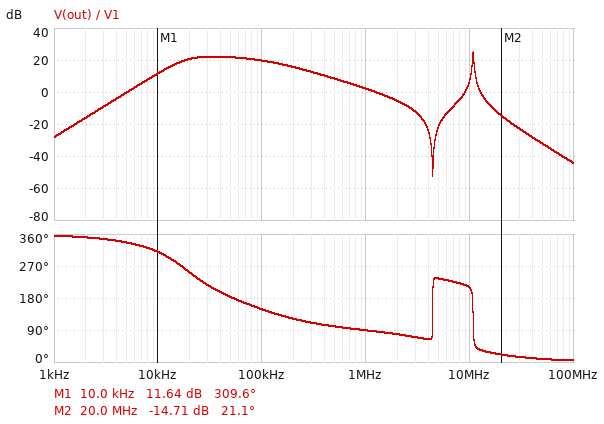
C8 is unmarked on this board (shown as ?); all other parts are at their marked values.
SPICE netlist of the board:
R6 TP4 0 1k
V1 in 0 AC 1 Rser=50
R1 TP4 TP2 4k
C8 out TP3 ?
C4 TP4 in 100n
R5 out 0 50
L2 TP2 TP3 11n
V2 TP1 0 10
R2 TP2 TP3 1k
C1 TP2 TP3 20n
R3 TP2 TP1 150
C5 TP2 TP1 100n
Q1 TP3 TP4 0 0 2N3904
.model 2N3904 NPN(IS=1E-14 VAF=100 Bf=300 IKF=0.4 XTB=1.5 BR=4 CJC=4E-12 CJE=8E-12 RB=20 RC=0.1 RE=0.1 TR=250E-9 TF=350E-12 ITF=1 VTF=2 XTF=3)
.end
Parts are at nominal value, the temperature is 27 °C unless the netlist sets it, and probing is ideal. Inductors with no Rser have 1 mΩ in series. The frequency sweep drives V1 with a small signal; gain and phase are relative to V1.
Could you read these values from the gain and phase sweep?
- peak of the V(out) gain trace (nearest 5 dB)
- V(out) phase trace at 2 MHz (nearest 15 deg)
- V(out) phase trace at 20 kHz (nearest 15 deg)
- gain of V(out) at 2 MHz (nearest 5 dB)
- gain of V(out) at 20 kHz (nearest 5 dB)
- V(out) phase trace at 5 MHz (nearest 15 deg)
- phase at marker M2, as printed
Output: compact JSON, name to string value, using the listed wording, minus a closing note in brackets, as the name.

{"peak of the V(out) gain trace": "25 dB", "V(out) phase trace at 2 MHz": "75 deg", "V(out) phase trace at 20 kHz": "255 deg", "gain of V(out) at 2 MHz": "-5 dB", "gain of V(out) at 20 kHz": "20 dB", "V(out) phase trace at 5 MHz": "240 deg", "phase at marker M2, as printed": "21.1 deg"}
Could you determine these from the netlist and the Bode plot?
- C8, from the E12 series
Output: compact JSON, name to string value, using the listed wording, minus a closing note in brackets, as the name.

{"C8, from the E12 series": "56 nF"}
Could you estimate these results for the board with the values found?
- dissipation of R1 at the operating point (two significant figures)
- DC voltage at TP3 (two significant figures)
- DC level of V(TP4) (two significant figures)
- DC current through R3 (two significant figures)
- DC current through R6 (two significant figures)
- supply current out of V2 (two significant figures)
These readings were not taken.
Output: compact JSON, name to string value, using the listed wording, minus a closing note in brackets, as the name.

{"dissipation of R1 at the operating point": "3.1 mW", "DC voltage at TP3": "4.3 V", "DC level of V(TP4)": "760 mV", "DC current through R3": "38 mA", "DC current through R6": "760 µA", "supply current out of V2": "38 mA"}
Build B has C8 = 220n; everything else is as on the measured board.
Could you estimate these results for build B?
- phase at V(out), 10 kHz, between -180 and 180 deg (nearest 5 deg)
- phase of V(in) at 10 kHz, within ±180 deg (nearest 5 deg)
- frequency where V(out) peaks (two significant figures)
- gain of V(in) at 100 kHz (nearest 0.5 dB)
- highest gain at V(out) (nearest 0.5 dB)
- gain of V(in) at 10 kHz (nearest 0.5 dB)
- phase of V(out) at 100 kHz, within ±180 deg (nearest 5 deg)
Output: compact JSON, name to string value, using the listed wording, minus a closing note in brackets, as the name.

{"phase at V(out), 10 kHz, between -180 and 180 deg": "-85 deg", "phase of V(in) at 10 kHz, within ±180 deg": "-15 deg", "frequency where V(out) peaks": "27 kHz", "gain of V(in) at 100 kHz": "-3.0 dB", "highest gain at V(out)": "25.5 dB", "gain of V(in) at 10 kHz": "-1.5 dB", "phase of V(out) at 100 kHz, within ±180 deg": "130 deg"}
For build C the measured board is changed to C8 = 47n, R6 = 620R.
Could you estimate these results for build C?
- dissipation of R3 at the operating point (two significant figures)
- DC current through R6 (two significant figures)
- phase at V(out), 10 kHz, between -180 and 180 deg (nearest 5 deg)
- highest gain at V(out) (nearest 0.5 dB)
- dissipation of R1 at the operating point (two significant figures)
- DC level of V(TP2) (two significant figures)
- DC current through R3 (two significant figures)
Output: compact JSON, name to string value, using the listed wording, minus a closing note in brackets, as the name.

{"dissipation of R3 at the operating point": "110 mW", "DC current through R6": "1.2 mA", "phase at V(out), 10 kHz, between -180 and 180 deg": "-55 deg", "highest gain at V(out)": "24.5 dB", "dissipation of R1 at the operating point": "6.6 mW", "DC level of V(TP2)": "5.9 V", "DC current through R3": "27 mA"}
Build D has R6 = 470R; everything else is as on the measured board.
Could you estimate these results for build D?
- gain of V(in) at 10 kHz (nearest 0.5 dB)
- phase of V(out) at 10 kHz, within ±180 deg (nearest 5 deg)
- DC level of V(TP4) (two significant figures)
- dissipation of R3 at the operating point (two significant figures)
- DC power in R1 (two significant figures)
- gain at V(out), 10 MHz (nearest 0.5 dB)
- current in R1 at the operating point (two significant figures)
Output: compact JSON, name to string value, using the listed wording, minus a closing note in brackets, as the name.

{"gain of V(in) at 10 kHz": "-1.5 dB", "phase of V(out) at 10 kHz, within ±180 deg": "-65 deg", "DC level of V(TP4)": "730 mV", "dissipation of R3 at the operating point": "53 mW", "DC power in R1": "10 mW", "gain at V(out), 10 MHz": "5.5 dB", "current in R1 at the operating point": "1.6 mA"}
